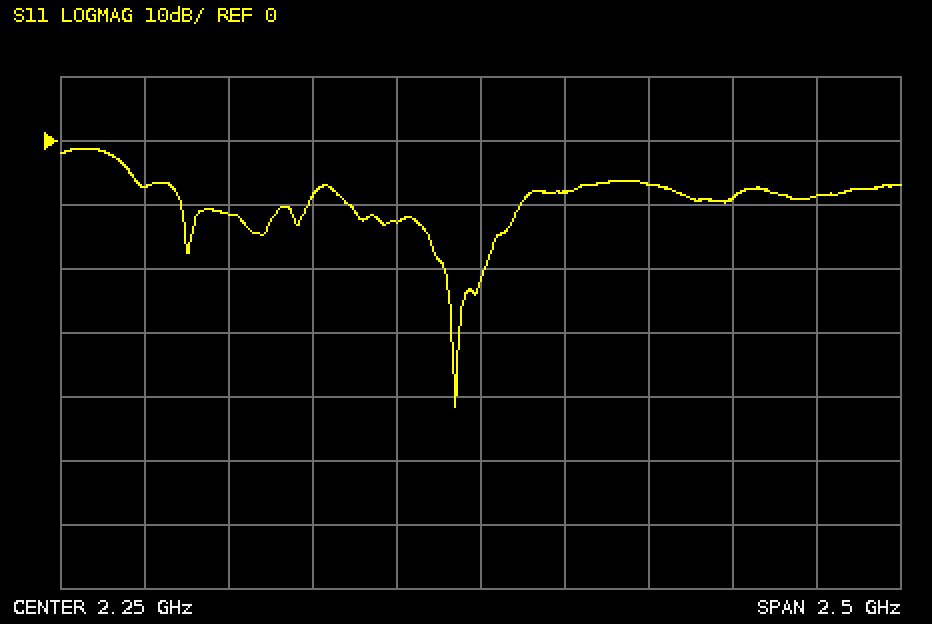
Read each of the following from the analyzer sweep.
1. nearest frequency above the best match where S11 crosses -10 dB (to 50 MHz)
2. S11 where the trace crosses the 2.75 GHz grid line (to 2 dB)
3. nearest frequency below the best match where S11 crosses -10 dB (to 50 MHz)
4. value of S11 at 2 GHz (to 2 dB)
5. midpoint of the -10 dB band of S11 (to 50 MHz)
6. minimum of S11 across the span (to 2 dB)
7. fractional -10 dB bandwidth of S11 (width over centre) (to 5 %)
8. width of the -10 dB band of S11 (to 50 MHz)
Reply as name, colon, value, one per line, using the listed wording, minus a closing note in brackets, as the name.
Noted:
nearest frequency above the best match where S11 crosses -10 dB: 2.35 GHz
S11 where the trace crosses the 2.75 GHz grid line: -6 dB
nearest frequency below the best match where S11 crosses -10 dB: 1.85 GHz
value of S11 at 2 GHz: -12 dB
midpoint of the -10 dB band of S11: 2.10 GHz
minimum of S11 across the span: -42 dB
fractional -10 dB bandwidth of S11 (width over centre): 25 %
width of the -10 dB band of S11: 500 MHz
